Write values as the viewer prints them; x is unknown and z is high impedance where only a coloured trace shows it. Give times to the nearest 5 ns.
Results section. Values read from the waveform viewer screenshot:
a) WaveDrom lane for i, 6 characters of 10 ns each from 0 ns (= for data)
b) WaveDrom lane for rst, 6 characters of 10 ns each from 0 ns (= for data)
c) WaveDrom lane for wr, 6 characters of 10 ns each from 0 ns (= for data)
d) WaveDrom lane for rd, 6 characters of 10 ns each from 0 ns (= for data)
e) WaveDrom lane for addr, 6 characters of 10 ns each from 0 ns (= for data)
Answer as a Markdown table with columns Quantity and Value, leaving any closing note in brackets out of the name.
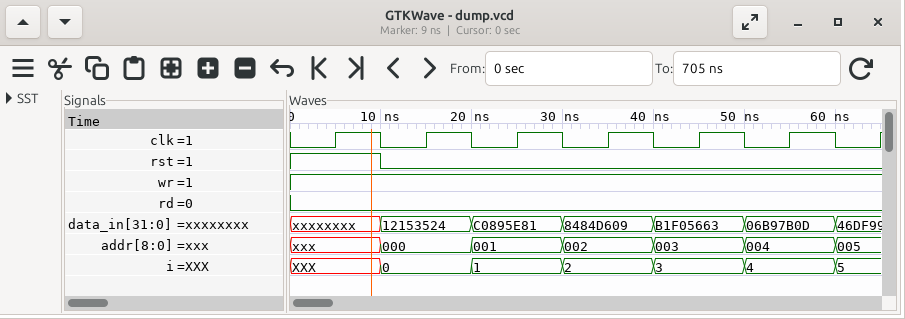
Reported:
| Quantity | Value |
|---|---|
| WaveDrom lane for i, 6 characters of 10 ns each from 0 ns | {name: 'i', wave: 'x=====', data: '0 1 2 3 4'} |
| WaveDrom lane for rst, 6 characters of 10 ns each from 0 ns | {name: 'rst', wave: '10....'} |
| WaveDrom lane for wr, 6 characters of 10 ns each from 0 ns | {name: 'wr', wave: '1.....'} |
| WaveDrom lane for rd, 6 characters of 10 ns each from 0 ns | {name: 'rd', wave: '0.....'} |
| WaveDrom lane for addr, 6 characters of 10 ns each from 0 ns | {name: 'addr', wave: 'x=====', data: '000 001 002 003 004'} |
